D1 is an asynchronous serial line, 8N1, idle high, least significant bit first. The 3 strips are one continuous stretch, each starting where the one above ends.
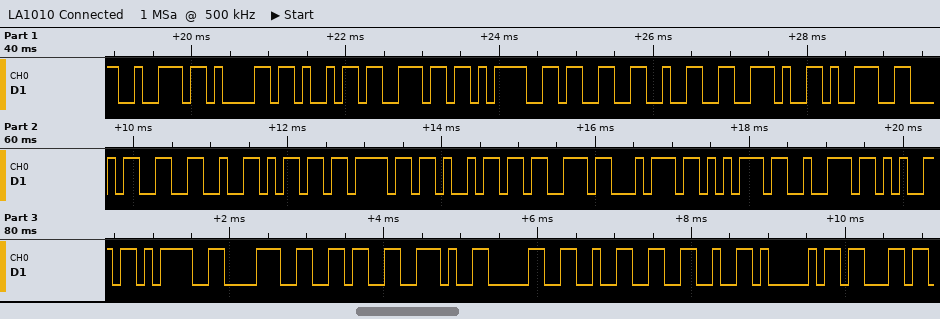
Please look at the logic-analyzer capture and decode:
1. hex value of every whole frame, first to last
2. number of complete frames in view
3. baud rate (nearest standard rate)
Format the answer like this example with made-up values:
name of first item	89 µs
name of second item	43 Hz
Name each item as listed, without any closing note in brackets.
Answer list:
hex value of every whole frame, first to last	72 61 69 6E 3D 33 32 2E 39 34 26 6D 6F 69 73 74 75 72 65 3D 38 36 2E 30 32 26 41 63
number of complete frames in view	28
baud rate	9600 baud
